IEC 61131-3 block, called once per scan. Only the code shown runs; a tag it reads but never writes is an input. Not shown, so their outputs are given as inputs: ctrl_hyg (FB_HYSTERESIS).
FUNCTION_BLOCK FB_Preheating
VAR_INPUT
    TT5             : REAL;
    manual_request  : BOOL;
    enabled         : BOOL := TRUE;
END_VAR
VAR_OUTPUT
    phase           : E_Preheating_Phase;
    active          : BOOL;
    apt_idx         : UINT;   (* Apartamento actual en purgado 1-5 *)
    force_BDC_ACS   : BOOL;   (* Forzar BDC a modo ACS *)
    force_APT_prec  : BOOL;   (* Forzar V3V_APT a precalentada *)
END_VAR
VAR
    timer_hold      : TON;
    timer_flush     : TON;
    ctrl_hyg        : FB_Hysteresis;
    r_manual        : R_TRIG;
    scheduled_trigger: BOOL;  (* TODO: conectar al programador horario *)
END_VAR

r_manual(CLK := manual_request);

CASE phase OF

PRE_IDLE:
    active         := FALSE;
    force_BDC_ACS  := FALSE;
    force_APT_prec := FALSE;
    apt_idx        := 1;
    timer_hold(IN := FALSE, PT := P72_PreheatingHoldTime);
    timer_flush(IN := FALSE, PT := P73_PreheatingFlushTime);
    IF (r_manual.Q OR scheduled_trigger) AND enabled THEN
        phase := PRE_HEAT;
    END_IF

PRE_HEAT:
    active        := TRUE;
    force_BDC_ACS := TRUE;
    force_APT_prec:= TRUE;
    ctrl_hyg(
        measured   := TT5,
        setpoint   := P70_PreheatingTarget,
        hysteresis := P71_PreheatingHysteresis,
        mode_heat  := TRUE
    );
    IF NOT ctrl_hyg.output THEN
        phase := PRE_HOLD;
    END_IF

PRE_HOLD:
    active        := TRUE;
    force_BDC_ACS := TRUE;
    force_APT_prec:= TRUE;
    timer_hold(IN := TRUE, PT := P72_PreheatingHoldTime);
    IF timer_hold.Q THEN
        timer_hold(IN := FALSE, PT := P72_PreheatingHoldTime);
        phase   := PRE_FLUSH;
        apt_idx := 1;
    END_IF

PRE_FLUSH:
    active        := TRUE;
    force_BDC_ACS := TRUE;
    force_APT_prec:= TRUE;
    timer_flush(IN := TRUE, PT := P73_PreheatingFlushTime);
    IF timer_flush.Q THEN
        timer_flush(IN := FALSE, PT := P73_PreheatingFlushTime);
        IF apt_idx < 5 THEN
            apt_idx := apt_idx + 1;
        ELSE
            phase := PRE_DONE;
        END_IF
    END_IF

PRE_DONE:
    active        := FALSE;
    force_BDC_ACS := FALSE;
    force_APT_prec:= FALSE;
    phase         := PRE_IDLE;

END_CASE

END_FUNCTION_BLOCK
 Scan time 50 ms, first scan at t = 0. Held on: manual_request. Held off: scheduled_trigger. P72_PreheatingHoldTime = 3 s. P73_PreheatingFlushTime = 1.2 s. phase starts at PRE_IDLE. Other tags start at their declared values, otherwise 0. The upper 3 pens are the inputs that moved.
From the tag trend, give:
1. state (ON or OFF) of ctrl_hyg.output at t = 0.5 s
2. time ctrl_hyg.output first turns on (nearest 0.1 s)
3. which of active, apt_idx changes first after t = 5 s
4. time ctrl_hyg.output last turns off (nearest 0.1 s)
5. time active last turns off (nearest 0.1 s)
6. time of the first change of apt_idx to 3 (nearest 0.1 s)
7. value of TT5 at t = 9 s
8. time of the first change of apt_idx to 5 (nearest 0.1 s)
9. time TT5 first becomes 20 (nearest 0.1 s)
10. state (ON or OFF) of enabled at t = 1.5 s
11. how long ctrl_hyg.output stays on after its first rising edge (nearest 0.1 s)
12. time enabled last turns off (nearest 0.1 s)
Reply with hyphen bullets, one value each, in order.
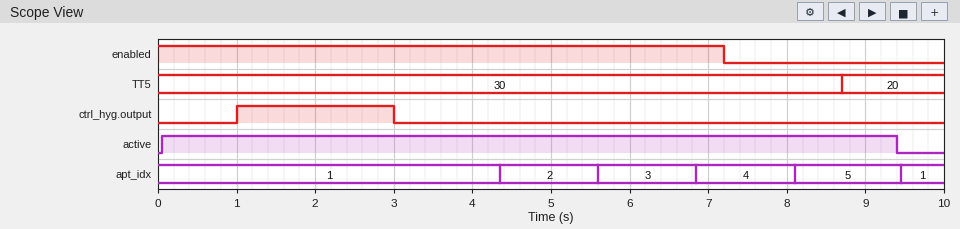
- OFF
- 1.0 s
- apt_idx
- 3.0 s
- 9.4 s
- 5.6 s
- 20
- 8.1 s
- 8.7 s
- ON
- 2.0 s
- 7.2 s
